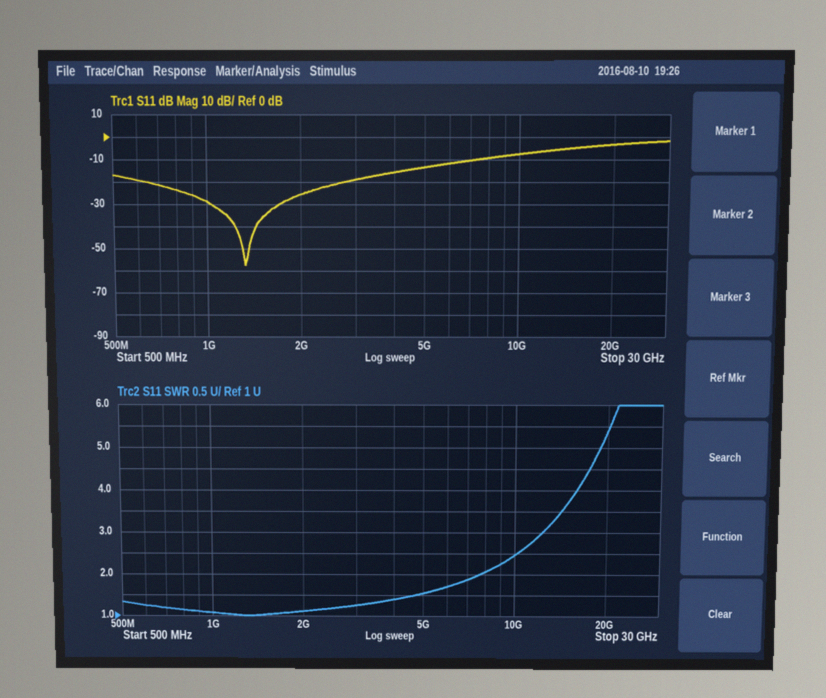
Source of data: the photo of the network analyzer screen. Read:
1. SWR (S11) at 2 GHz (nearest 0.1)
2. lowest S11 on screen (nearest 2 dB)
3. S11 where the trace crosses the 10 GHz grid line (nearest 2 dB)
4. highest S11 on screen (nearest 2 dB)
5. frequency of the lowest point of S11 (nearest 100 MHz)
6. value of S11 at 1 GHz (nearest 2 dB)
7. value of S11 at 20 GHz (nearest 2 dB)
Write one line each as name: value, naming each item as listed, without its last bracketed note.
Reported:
SWR (S11) at 2 GHz: 1.1
lowest S11 on screen: -58 dB
S11 where the trace crosses the 10 GHz grid line: -8 dB
highest S11 on screen: -2 dB
frequency of the lowest point of S11: 1.3 GHz
value of S11 at 1 GHz: -28 dB
value of S11 at 20 GHz: -4 dB
